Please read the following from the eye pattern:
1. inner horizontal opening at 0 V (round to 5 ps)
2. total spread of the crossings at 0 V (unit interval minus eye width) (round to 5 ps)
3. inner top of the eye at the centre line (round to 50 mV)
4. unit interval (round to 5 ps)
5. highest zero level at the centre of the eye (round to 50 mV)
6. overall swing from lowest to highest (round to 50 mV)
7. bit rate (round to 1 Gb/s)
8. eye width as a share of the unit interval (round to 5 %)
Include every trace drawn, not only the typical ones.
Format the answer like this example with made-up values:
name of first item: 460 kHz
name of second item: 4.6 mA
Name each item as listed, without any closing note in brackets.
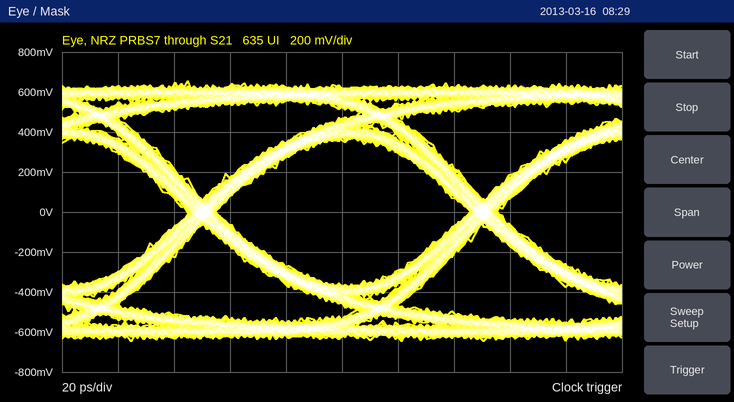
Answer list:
inner horizontal opening at 0 V: 90 ps
total spread of the crossings at 0 V (unit interval minus eye width): 10 ps
inner top of the eye at the centre line: 350 mV
unit interval: 100 ps
highest zero level at the centre of the eye: -350 mV
overall swing from lowest to highest: 1.30 V
bit rate: 10 Gb/s
eye width as a share of the unit interval: 90 %
